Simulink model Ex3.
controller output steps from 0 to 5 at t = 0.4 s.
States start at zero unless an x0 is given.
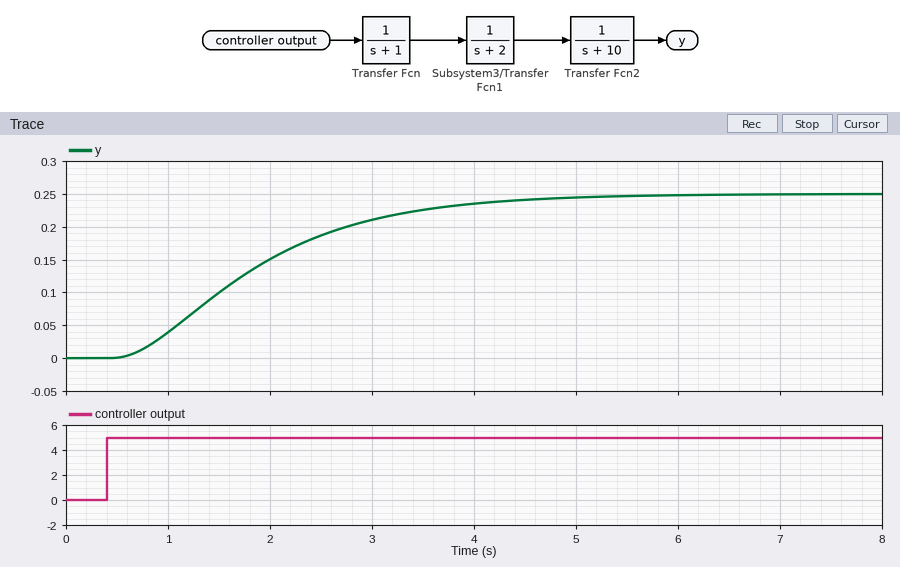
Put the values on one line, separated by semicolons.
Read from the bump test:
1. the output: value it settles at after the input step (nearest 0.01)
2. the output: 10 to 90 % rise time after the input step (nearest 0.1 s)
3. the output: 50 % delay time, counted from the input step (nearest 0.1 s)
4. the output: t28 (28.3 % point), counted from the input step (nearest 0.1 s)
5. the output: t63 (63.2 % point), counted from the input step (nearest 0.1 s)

0.25; 2.6 s; 1.3 s; 0.9 s; 1.7 s
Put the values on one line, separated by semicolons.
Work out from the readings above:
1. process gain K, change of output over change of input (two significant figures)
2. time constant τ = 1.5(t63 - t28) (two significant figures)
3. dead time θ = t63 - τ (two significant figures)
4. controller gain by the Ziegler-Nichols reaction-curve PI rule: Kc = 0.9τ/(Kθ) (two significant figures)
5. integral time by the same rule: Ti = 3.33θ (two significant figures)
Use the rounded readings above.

0.050; 1.2 s; 0.50 s; 43; 1.7 s
